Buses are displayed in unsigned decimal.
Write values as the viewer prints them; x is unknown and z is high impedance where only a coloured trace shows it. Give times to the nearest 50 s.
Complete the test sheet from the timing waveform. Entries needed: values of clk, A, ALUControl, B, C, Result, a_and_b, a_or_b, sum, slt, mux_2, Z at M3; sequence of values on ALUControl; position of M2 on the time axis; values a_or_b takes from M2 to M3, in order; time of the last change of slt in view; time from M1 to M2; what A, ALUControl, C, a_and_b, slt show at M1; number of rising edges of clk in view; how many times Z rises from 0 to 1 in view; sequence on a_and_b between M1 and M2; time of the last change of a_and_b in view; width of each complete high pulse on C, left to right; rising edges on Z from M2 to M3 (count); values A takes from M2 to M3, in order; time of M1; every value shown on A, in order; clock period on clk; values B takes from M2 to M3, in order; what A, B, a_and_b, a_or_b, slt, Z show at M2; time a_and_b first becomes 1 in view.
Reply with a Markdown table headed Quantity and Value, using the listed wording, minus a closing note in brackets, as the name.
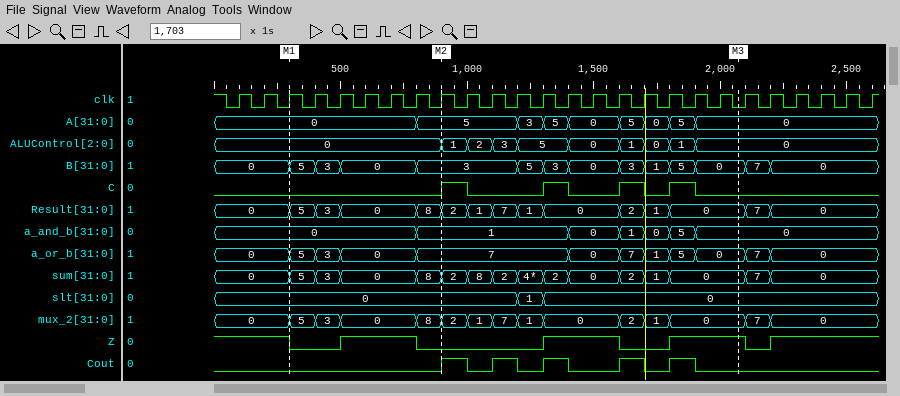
| Quantity | Value |
|---|---|
| values of clk, A, ALUControl, B, C, Result, a_and_b, a_or_b, sum, slt, mux_2, Z at M3 | clk=0, A=0, ALUControl=0, B=0, C=0, Result=0, a_and_b=0, a_or_b=0, sum=0, slt=0, mux_2=0, Z=1 |
| sequence of values on ALUControl | 0, 1, 2, 3, 5, 0, 1, 0, 1, 0 |
| position of M2 on the time axis | 900 s |
| values a_or_b takes from M2 to M3, in order | 7, 0, 7, 1, 5, 0 |
| time of the last change of slt in view | 1300 s |
| time from M1 to M2 | 600 s |
| what A, ALUControl, C, a_and_b, slt show at M1 | A=0, ALUControl=0, C=0, a_and_b=0, slt=0 |
| number of rising edges of clk in view | 26 |
| how many times Z rises from 0 to 1 in view | 4 |
| sequence on a_and_b between M1 and M2 | 0, 1 |
| time of the last change of a_and_b in view | 1900 s |
| width of each complete high pulse on C, left to right | 100 s, 100 s, 100 s, 100 s |
| rising edges on Z from M2 to M3 | 2 |
| values A takes from M2 to M3, in order | 5, 3, 5, 0, 5, 0, 5, 0 |
| time of M1 | 300 s |
| every value shown on A, in order | 0, 5, 3, 5, 0, 5, 0, 5, 0 |
| clock period on clk | 100 s |
| values B takes from M2 to M3, in order | 3, 5, 3, 0, 3, 1, 5, 0 |
| what A, B, a_and_b, a_or_b, slt, Z show at M2 | A=5, B=3, a_and_b=1, a_or_b=7, slt=0, Z=0 |
| time a_and_b first becomes 1 in view | 800 s |
